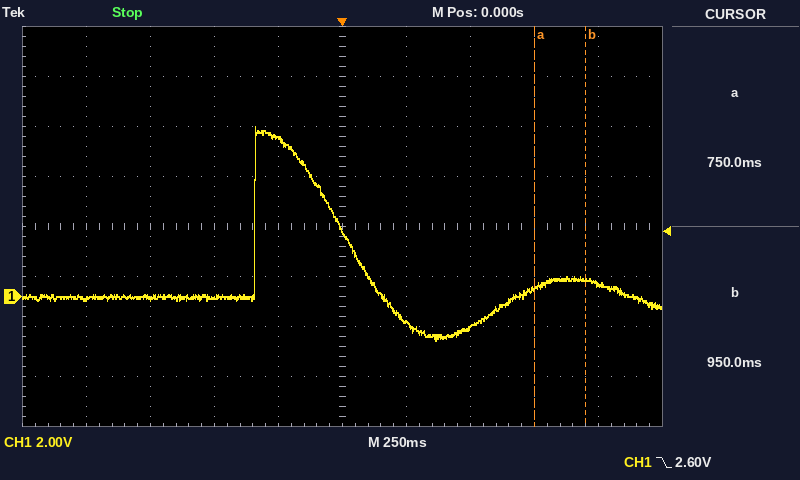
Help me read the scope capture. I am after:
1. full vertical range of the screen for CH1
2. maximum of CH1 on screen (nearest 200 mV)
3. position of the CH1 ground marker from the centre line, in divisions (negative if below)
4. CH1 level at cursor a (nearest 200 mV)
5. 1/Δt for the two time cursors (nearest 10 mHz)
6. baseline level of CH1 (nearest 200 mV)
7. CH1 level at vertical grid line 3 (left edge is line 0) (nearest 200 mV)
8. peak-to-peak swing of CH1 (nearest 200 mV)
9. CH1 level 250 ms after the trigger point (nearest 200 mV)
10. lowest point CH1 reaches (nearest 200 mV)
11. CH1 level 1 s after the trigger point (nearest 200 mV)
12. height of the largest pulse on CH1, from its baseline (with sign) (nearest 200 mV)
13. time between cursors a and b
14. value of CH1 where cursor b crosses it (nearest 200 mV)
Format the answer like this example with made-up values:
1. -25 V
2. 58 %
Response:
1. 16 V
2. 6.8 V
3. -1.4 div
4. 400 mV
5. 5.00 Hz
6. 0.0 V
7. 0.0 V
8. 8.6 V
9. -1.0 V
10. -1.8 V
11. 600 mV
12. +6.8 V
13. 200 ms
14. 600 mV
